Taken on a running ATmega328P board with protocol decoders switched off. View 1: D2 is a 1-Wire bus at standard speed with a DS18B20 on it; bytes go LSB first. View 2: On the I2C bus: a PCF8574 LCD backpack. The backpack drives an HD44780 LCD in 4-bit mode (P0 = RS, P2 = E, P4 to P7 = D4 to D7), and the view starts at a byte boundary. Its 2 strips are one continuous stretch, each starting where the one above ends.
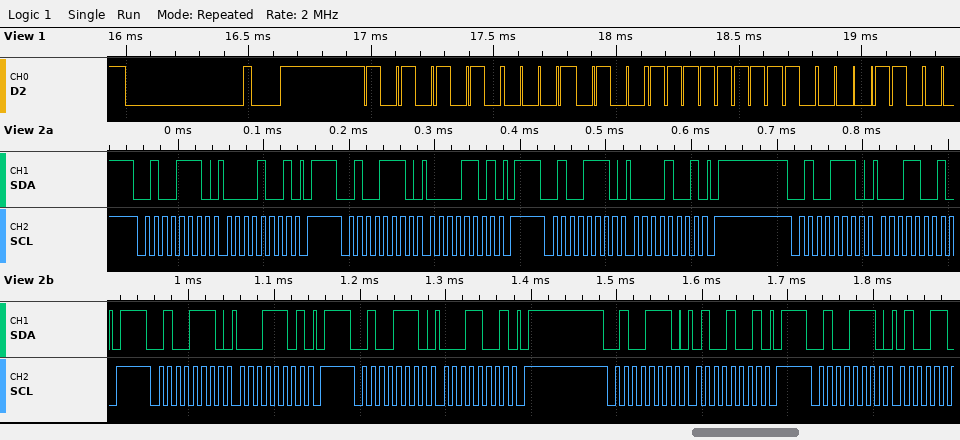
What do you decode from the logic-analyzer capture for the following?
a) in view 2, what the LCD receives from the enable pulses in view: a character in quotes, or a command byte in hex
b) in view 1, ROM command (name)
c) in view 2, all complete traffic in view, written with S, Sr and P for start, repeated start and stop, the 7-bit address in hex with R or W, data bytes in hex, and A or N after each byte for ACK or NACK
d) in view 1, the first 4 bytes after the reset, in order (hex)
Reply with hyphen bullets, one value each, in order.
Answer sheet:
- data 0x01
- Match ROM
- S 27W A 09 A P S 27W A 0D A P S 27W A 09 A P S 27W A 19 A P S 27W A 1D A P S 27W A 19 A P S 27W A 49 A P S 27W A
- 55 28 FF 61
